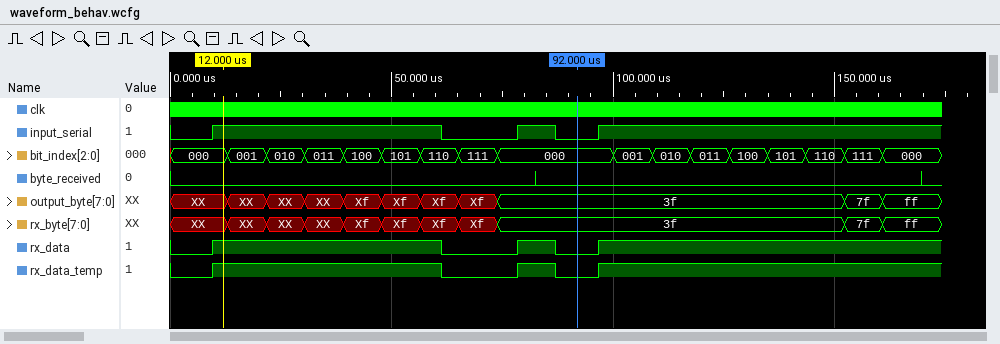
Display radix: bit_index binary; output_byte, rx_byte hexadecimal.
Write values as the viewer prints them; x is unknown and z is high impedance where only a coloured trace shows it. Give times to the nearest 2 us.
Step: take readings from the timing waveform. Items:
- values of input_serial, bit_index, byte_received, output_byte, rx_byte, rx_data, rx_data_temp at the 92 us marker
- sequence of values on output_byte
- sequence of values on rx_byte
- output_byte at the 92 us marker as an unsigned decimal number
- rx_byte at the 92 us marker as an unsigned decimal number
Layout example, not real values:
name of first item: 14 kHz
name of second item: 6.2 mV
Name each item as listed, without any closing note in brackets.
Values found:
values of input_serial, bit_index, byte_received, output_byte, rx_byte, rx_data, rx_data_temp at the 92 us marker: input_serial=0, bit_index=000, byte_received=0, output_byte=3f, rx_byte=3f, rx_data=0, rx_data_temp=0
sequence of values on output_byte: XX, XX, XX, XX, Xf, Xf, Xf, Xf, 3f, 7f, ff
sequence of values on rx_byte: XX, XX, XX, XX, Xf, Xf, Xf, Xf, 3f, 7f, ff
output_byte at the 92 us marker as an unsigned decimal number: 63
rx_byte at the 92 us marker as an unsigned decimal number: 63
